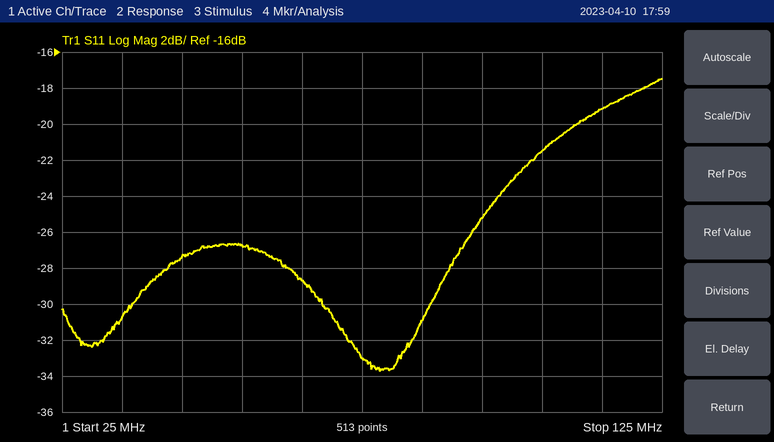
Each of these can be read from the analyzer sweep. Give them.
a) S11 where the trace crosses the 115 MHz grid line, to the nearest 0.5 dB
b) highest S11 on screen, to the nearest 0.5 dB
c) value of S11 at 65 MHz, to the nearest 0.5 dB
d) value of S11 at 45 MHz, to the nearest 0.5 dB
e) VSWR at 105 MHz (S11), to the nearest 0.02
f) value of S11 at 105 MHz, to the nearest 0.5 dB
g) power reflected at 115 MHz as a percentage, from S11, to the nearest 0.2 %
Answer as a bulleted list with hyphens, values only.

- -19.0 dB
- -17.5 dB
- -28.5 dB
- -27.5 dB
- 1.18
- -21.5 dB
- 1.2 %
